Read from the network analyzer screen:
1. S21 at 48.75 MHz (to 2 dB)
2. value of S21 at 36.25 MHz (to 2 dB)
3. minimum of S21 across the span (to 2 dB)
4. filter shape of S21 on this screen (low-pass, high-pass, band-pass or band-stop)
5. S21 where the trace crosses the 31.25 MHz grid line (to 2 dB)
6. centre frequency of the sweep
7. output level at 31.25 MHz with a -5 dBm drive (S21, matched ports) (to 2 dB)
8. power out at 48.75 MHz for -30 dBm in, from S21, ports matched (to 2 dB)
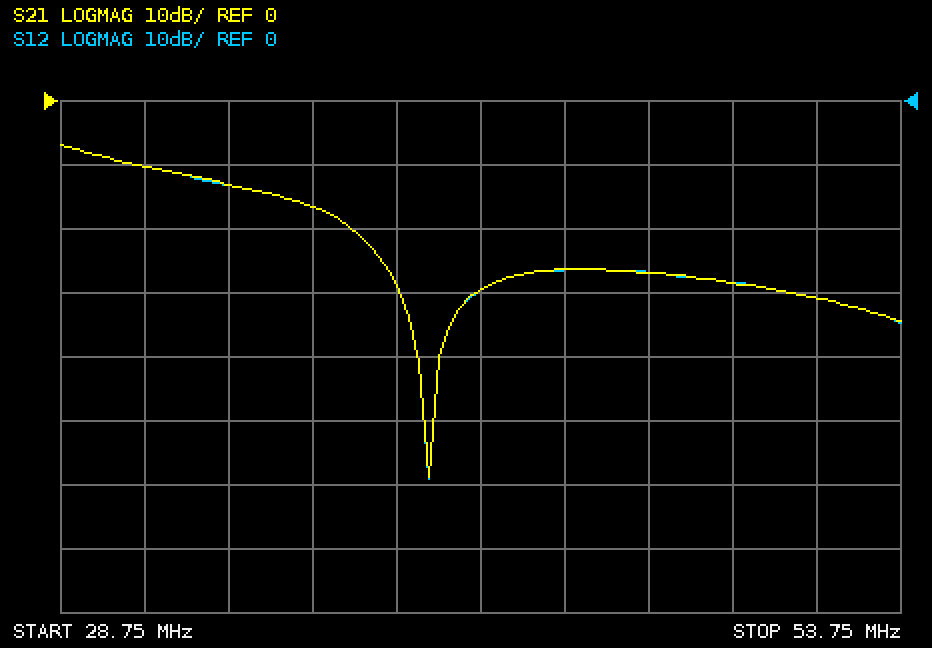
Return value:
-28 dB
-16 dB
-58 dB
low-pass
-10 dB
41.25 MHz
-16 dBm
-58 dBm
